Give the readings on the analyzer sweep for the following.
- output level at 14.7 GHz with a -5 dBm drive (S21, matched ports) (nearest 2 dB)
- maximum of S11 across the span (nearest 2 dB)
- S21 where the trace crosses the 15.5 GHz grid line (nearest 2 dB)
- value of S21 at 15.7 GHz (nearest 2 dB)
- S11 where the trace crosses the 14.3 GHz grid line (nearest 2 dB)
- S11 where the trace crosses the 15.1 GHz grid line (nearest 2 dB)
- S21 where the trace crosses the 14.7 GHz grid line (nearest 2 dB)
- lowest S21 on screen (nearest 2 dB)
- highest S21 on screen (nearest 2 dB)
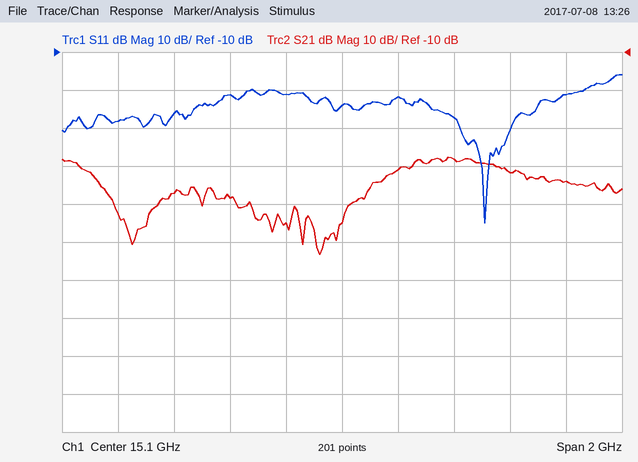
-54 dBm
-16 dB
-38 dB
-42 dB
-28 dB
-24 dB
-48 dB
-64 dB
-38 dB
